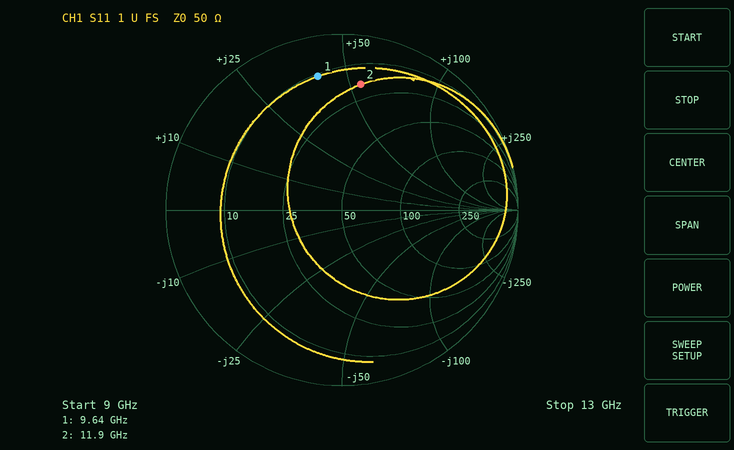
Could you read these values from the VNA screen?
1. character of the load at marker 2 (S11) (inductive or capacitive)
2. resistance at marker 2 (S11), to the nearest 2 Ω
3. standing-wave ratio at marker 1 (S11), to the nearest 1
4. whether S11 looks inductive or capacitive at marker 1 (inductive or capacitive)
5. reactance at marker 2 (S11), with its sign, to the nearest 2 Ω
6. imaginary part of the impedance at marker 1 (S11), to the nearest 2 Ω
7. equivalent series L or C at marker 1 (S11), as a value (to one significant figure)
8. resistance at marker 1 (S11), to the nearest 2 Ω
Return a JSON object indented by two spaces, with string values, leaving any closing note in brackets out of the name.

{
  "character of the load at marker 2 (S11)": "inductive",
  "resistance at marker 2 (S11), to the nearest 2 Ω": "18 Ω",
  "standing-wave ratio at marker 1 (S11), to the nearest 1": "8",
  "whether S11 looks inductive or capacitive at marker 1": "inductive",
  "reactance at marker 2 (S11), with its sign, to the nearest 2 Ω": "+54 Ω",
  "imaginary part of the impedance at marker 1 (S11), to the nearest 2 Ω": "+40 Ω",
  "equivalent series L or C at marker 1 (S11), as a value": "700 pH",
  "resistance at marker 1 (S11), to the nearest 2 Ω": "10 Ω"
}
